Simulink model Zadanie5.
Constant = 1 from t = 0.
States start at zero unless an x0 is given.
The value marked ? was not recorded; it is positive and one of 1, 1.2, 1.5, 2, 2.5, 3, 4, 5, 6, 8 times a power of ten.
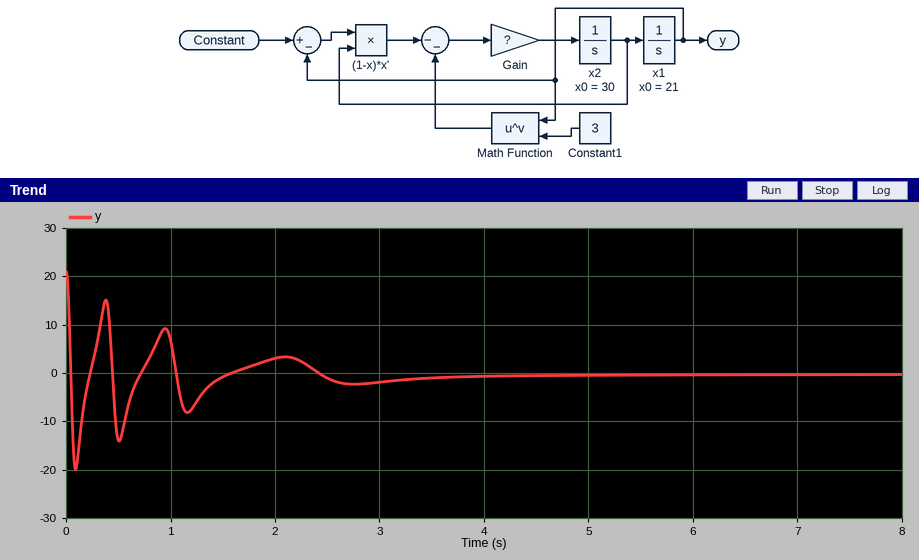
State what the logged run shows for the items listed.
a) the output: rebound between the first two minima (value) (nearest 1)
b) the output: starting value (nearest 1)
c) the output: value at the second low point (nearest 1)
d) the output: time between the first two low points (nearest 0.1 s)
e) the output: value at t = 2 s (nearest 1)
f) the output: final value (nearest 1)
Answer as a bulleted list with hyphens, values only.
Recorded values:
- 15
- 21
- -14
- 0.4 s
- 3
- 0
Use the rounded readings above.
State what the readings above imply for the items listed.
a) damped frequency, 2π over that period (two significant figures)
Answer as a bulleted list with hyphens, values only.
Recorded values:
- 16 rad/s
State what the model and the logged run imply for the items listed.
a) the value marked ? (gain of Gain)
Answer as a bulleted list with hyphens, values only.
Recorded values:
- 2
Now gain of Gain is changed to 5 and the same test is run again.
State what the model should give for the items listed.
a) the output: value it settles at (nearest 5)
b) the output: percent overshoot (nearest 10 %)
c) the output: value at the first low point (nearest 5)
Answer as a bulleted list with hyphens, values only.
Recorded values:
- 0
- 90 %
- -20
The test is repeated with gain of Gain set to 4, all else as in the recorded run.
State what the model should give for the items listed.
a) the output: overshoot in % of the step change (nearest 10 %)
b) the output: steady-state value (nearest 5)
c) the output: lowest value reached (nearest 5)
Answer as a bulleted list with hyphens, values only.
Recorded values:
- 90 %
- 0
- -20
